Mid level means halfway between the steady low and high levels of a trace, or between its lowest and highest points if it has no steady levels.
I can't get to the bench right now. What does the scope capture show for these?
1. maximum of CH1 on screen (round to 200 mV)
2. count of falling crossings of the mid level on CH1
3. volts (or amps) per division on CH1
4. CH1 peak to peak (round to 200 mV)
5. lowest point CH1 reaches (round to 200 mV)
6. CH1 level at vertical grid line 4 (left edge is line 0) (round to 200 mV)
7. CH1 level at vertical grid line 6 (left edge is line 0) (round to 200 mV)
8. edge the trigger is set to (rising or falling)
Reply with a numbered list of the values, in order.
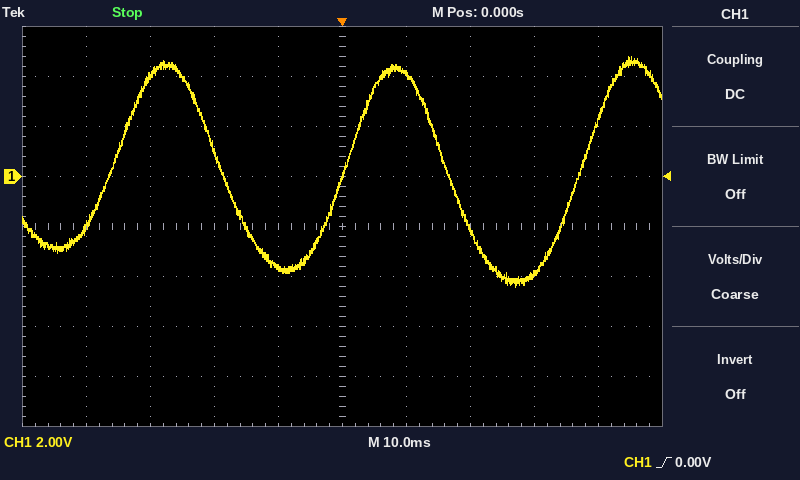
1. 4.8 V
2. 2
3. 2 V
4. 9.2 V
5. -4.4 V
6. -3.6 V
7. 4.0 V
8. rising
